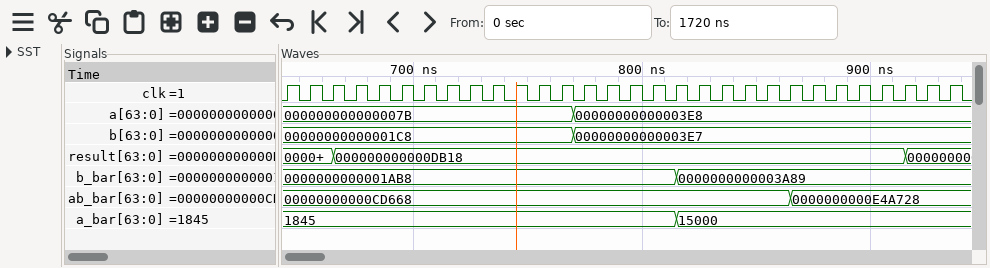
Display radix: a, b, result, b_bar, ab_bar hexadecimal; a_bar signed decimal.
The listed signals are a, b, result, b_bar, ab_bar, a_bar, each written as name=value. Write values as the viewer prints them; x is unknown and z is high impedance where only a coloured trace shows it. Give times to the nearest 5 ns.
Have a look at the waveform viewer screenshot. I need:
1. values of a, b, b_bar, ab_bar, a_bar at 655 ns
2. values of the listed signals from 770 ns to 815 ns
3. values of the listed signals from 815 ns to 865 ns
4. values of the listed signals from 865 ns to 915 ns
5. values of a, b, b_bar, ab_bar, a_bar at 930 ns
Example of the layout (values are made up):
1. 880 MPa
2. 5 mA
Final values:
1. a=000000000000007B, b=00000000000001C8, b_bar=0000000000001AB8, ab_bar=00000000000CD668, a_bar=1845
2. a=00000000000003E8, b=00000000000003E7, result=000000000000DB18, b_bar=0000000000001AB8, ab_bar=00000000000CD668, a_bar=1845
3. a=00000000000003E8, b=00000000000003E7, result=000000000000DB18, b_bar=0000000000003A89, ab_bar=00000000000CD668, a_bar=15000
4. a=00000000000003E8, b=00000000000003E7, result=000000000000DB18, b_bar=0000000000003A89, ab_bar=0000000000E4A728, a_bar=15000
5. a=00000000000003E8, b=00000000000003E7, b_bar=0000000000003A89, ab_bar=0000000000E4A728, a_bar=15000
